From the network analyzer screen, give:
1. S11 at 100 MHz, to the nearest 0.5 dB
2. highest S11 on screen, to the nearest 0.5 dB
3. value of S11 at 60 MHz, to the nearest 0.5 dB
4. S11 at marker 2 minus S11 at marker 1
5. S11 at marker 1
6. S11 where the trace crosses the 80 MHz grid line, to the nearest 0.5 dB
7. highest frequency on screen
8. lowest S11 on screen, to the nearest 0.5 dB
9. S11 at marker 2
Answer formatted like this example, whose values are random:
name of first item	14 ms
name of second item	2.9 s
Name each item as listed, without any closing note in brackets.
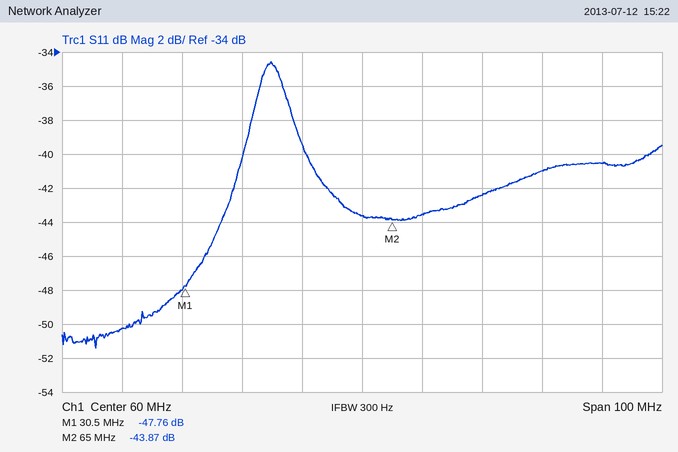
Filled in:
S11 at 100 MHz, to the nearest 0.5 dB	-40.5 dB
highest S11 on screen, to the nearest 0.5 dB	-34.5 dB
value of S11 at 60 MHz, to the nearest 0.5 dB	-43.5 dB
S11 at marker 2 minus S11 at marker 1	3.89 dB
S11 at marker 1	-47.76 dB
S11 where the trace crosses the 80 MHz grid line, to the nearest 0.5 dB	-42.5 dB
highest frequency on screen	110 MHz
lowest S11 on screen, to the nearest 0.5 dB	-51.5 dB
S11 at marker 2	-43.87 dB
